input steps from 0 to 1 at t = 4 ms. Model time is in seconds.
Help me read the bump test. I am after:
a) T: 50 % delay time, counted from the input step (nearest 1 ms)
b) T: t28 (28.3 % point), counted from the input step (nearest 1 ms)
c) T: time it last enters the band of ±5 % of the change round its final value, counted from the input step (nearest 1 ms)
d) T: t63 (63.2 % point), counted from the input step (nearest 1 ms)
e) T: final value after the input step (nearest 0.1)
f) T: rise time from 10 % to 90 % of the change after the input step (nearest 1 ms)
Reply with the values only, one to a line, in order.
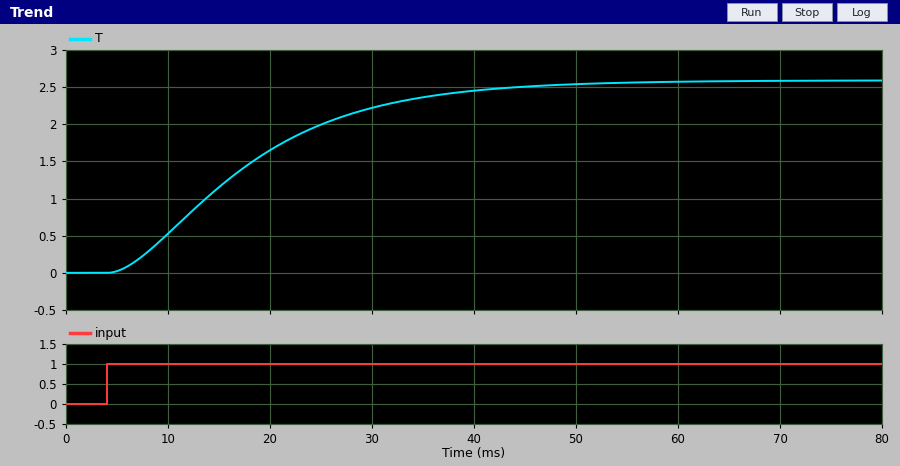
12 ms
8 ms
37 ms
16 ms
2.6
26 ms
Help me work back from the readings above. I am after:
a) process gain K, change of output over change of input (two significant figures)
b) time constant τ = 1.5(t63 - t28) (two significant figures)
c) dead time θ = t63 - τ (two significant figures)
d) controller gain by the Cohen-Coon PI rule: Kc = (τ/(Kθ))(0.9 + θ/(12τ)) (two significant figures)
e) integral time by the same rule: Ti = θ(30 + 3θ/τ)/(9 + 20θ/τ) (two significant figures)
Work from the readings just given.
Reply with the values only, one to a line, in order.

2.6
12 ms
4.0 ms
1.1
7.9 ms
